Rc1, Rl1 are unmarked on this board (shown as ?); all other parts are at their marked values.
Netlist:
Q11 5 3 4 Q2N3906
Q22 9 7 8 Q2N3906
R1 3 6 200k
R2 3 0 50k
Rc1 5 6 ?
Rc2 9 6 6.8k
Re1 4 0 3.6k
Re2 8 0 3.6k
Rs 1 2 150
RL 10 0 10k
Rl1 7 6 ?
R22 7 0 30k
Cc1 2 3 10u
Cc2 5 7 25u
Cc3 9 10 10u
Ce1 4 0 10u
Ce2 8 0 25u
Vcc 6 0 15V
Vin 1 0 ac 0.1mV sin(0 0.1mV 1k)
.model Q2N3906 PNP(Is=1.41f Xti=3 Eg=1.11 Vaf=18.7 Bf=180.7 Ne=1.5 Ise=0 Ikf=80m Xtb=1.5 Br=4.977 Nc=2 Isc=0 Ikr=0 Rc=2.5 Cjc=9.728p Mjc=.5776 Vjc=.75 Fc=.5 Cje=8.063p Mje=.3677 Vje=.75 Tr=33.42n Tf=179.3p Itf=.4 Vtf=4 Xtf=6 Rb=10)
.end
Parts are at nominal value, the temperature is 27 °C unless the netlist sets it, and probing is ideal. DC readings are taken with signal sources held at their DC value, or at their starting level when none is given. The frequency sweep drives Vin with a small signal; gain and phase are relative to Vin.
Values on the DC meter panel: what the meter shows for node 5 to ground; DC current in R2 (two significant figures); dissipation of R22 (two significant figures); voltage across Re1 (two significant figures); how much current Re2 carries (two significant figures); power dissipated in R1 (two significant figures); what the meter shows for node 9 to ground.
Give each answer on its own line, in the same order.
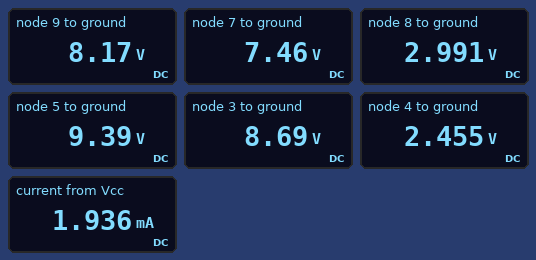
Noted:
9.39 V
170 µA
1.9 mW
2.5 V
830 µA
200 µW
8.17 V
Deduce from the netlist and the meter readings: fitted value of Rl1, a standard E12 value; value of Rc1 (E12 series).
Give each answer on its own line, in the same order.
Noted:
100 kΩ
6.8 kΩ
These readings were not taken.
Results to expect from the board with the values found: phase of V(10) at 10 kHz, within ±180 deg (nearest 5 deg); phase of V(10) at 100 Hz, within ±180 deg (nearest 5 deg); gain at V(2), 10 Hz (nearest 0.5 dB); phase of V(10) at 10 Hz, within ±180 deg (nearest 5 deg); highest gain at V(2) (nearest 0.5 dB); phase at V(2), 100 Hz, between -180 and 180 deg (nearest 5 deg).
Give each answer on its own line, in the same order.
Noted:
0 deg
0 deg
0 dB
20 deg
0 dB
0 deg
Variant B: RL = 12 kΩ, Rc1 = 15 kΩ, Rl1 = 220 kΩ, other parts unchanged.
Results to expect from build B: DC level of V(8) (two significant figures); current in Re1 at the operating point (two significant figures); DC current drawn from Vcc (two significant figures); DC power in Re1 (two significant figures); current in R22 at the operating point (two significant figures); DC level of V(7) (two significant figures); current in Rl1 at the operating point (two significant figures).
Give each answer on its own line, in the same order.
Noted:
3.3 V
430 µA
1.7 mA
660 µW
230 µA
6.8 V
37 µA
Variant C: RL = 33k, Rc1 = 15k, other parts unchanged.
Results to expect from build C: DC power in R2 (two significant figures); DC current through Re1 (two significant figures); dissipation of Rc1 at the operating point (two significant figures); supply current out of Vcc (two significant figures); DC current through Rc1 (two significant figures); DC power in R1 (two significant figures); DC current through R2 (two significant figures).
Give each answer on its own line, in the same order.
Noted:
860 µW
430 µA
4.0 mW
1.6 mA
520 µA
360 µW
130 µA
